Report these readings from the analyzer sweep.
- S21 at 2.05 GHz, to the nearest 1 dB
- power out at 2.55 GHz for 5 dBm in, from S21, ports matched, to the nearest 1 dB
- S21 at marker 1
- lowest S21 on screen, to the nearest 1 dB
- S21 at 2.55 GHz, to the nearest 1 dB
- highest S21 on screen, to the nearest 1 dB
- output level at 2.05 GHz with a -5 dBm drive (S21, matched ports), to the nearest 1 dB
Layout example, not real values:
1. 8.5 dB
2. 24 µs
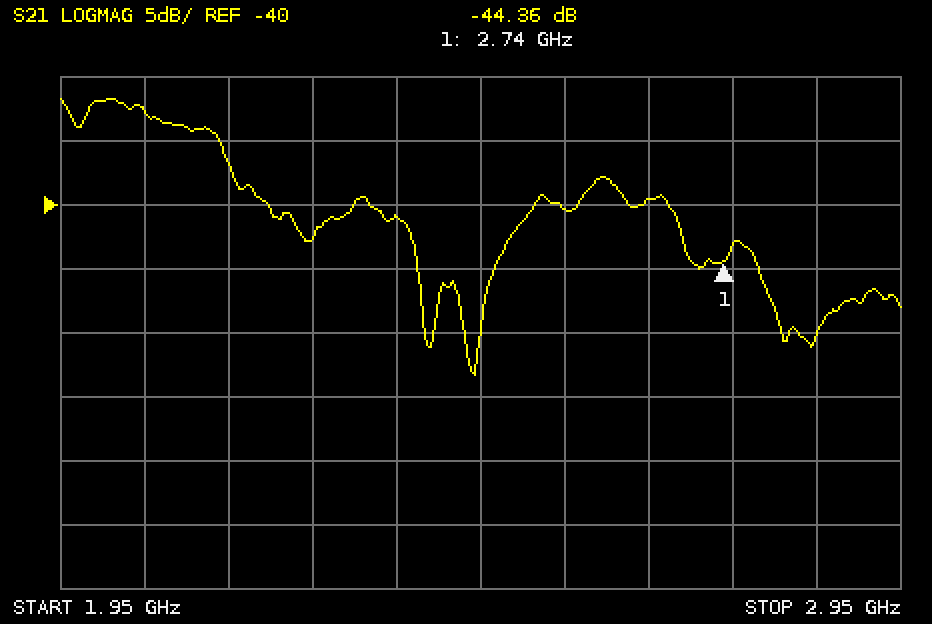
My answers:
1. -33 dB
2. -35 dBm
3. -44.36 dB
4. -53 dB
5. -40 dB
6. -32 dB
7. -38 dBm
